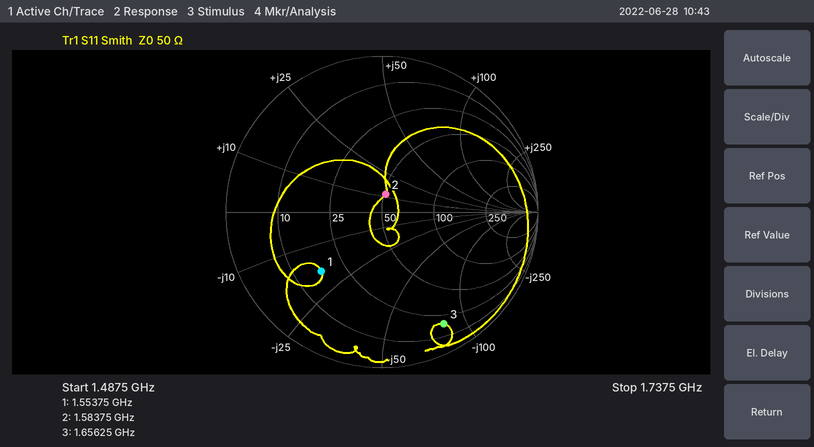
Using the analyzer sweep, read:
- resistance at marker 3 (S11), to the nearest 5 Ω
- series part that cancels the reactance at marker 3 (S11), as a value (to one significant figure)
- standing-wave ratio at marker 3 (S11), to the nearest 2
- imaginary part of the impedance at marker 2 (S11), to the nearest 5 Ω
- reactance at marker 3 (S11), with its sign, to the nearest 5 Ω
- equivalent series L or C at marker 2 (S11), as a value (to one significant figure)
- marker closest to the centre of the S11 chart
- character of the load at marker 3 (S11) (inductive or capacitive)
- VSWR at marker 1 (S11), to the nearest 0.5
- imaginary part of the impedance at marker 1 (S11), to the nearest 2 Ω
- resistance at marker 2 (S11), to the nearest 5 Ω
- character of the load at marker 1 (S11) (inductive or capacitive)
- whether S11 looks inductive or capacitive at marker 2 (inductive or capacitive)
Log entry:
20 Ω
8 nH
10
+10 Ω
-80 Ω
1 nH
marker 2
capacitive
3.5
-18 Ω
50 Ω
capacitive
inductive
